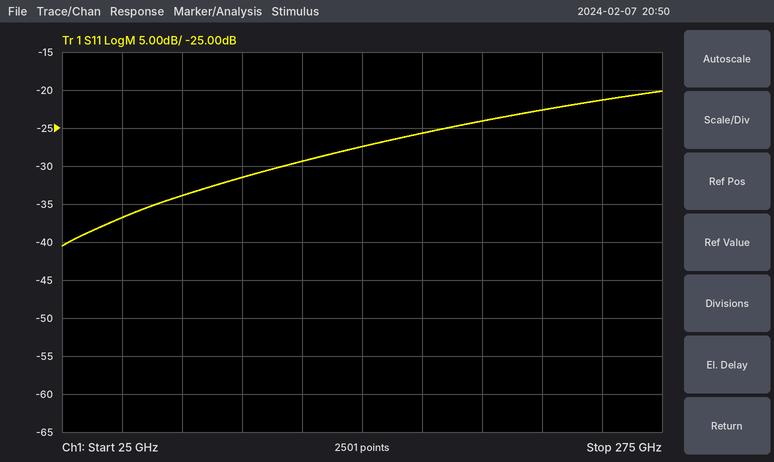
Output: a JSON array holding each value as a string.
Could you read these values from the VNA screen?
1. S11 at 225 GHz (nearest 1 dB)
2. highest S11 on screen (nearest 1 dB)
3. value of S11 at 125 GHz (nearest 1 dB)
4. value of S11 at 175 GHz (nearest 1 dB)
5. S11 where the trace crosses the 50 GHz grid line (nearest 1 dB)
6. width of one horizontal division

["-23 dB", "-20 dB", "-29 dB", "-26 dB", "-37 dB", "25 GHz"]
